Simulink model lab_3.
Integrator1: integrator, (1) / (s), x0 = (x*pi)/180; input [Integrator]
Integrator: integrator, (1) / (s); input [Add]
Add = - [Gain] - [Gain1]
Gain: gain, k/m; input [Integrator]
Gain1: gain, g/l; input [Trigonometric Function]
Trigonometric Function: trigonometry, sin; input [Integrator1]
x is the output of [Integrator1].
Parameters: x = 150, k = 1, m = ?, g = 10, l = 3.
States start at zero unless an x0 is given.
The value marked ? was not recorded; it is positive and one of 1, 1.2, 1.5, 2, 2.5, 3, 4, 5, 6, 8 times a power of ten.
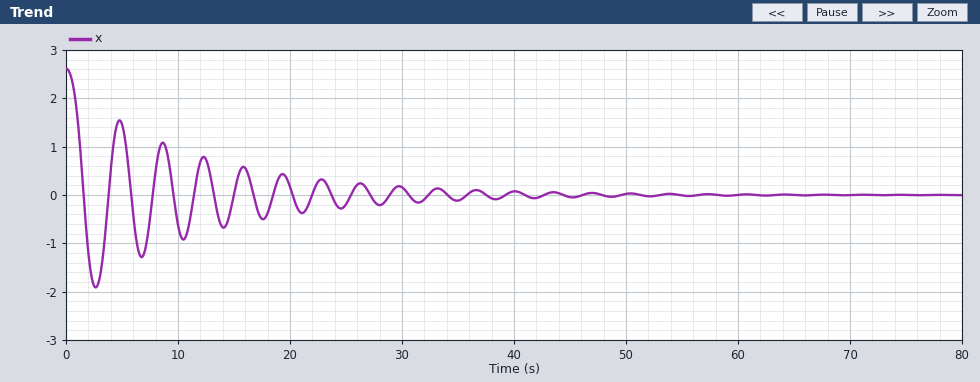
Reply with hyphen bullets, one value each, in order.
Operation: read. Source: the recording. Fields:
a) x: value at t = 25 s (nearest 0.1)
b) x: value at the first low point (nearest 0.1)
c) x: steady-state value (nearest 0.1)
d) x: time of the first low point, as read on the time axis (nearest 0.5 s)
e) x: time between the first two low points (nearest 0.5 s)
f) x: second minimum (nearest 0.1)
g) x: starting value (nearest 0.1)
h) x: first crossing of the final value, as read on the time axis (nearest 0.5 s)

- -0.2
- -1.9
- 0.0
- 2.5 s
- 4.0 s
- -1.3
- 2.6
- 1.5 s
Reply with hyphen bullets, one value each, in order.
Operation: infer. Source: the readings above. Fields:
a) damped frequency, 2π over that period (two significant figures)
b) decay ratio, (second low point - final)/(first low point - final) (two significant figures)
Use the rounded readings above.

- 1.6 rad/s
- 0.68
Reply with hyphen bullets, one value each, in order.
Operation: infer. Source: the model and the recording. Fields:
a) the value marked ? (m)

- 6
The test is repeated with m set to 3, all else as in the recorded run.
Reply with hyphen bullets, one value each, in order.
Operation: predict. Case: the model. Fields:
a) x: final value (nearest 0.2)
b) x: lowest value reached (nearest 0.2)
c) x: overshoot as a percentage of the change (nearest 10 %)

- 0.0
- -1.6
- 60 %
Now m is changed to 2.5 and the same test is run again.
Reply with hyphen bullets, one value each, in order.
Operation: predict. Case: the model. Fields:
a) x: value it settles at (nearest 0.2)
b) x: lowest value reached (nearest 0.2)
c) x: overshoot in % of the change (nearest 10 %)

- 0.0
- -1.4
- 50 %
